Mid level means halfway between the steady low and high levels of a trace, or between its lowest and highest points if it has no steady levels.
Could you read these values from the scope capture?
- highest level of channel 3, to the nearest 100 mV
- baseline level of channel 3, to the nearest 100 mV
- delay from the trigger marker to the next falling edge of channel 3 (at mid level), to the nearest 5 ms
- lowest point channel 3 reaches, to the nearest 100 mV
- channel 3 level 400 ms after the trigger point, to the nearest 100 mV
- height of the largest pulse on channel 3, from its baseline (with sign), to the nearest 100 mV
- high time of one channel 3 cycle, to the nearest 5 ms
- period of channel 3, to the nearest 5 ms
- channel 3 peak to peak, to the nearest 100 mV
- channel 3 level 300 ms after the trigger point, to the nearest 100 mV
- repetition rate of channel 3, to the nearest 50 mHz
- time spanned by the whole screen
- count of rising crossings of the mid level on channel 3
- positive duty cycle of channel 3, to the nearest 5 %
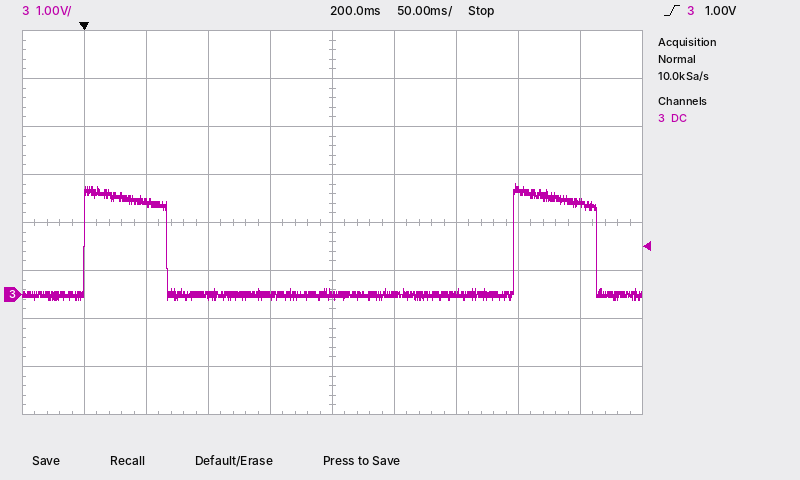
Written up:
2.3 V
0.0 V
65 ms
-100 mV
1.9 V
+2.3 V
65 ms
345 ms
2.4 V
0.0 V
2.90 Hz
500 ms
2
20 %
